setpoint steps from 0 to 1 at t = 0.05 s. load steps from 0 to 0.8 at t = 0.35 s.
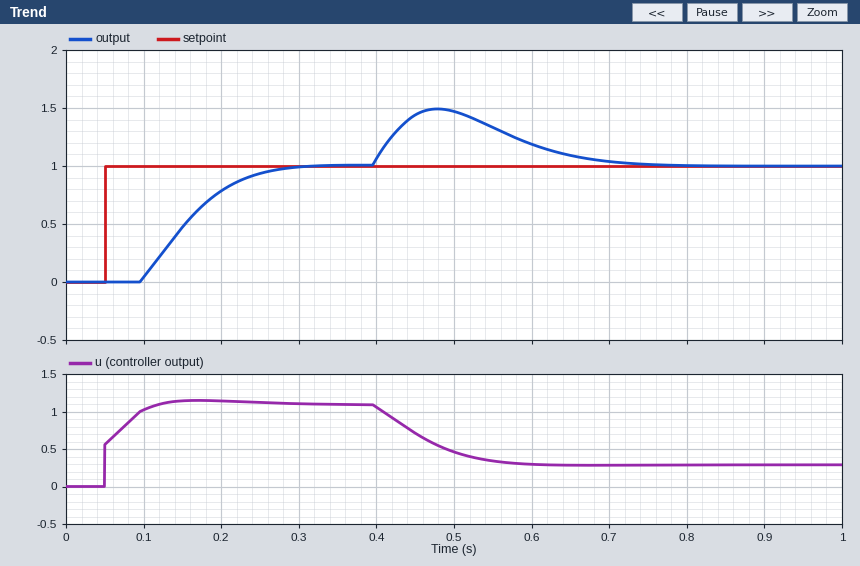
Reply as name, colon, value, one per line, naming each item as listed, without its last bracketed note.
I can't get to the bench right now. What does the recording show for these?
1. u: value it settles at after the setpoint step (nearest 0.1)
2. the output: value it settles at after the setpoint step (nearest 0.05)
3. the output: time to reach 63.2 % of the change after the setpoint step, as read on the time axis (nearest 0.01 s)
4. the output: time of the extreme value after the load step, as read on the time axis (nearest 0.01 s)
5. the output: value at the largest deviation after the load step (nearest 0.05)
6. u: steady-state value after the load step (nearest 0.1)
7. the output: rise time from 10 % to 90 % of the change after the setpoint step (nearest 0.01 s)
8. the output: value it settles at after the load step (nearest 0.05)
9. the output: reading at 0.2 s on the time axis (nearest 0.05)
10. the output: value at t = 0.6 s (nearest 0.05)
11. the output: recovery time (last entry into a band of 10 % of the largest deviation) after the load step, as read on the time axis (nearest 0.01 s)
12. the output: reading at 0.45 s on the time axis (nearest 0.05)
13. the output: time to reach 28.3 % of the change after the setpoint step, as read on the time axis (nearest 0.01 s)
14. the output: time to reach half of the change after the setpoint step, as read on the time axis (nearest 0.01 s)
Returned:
u: value it settles at after the setpoint step: 1.1
the output: value it settles at after the setpoint step: 1.00
the output: time to reach 63.2 % of the change after the setpoint step, as read on the time axis: 0.17 s
the output: time of the extreme value after the load step, as read on the time axis: 0.48 s
the output: value at the largest deviation after the load step: 1.50
u: steady-state value after the load step: 0.3
the output: rise time from 10 % to 90 % of the change after the setpoint step: 0.13 s
the output: value it settles at after the load step: 1.00
the output: reading at 0.2 s on the time axis: 0.80
the output: value at t = 0.6 s: 1.20
the output: recovery time (last entry into a band of 10 % of the largest deviation) after the load step, as read on the time axis: 0.69 s
the output: reading at 0.45 s on the time axis: 1.45
the output: time to reach 28.3 % of the change after the setpoint step, as read on the time axis: 0.13 s
the output: time to reach half of the change after the setpoint step, as read on the time axis: 0.15 s
